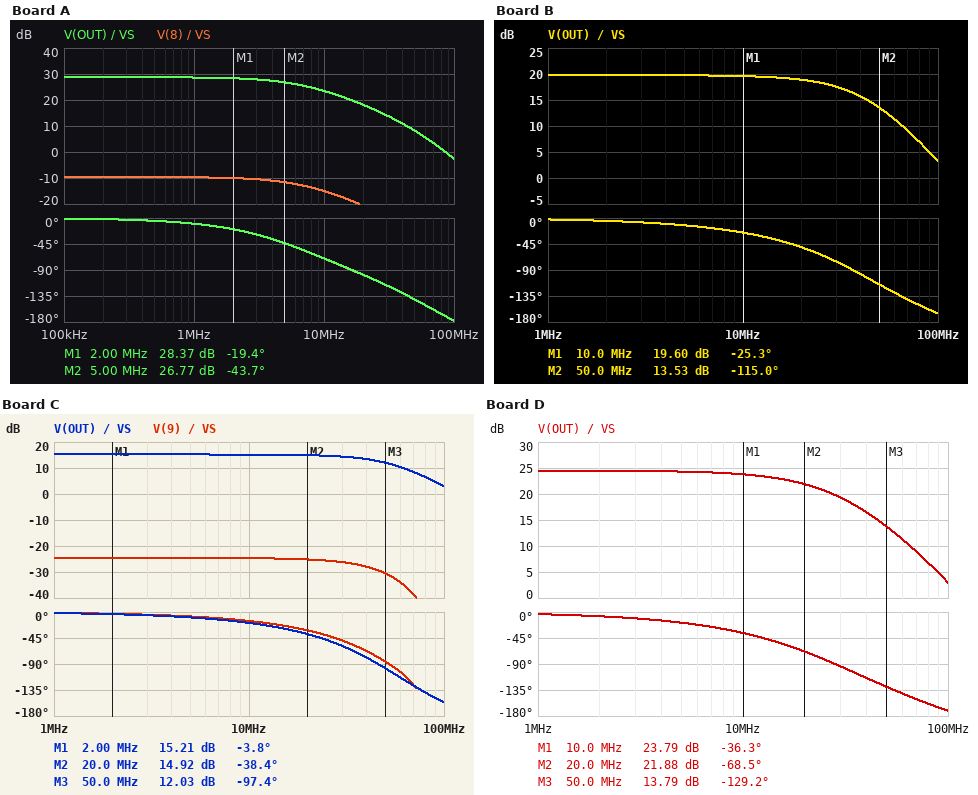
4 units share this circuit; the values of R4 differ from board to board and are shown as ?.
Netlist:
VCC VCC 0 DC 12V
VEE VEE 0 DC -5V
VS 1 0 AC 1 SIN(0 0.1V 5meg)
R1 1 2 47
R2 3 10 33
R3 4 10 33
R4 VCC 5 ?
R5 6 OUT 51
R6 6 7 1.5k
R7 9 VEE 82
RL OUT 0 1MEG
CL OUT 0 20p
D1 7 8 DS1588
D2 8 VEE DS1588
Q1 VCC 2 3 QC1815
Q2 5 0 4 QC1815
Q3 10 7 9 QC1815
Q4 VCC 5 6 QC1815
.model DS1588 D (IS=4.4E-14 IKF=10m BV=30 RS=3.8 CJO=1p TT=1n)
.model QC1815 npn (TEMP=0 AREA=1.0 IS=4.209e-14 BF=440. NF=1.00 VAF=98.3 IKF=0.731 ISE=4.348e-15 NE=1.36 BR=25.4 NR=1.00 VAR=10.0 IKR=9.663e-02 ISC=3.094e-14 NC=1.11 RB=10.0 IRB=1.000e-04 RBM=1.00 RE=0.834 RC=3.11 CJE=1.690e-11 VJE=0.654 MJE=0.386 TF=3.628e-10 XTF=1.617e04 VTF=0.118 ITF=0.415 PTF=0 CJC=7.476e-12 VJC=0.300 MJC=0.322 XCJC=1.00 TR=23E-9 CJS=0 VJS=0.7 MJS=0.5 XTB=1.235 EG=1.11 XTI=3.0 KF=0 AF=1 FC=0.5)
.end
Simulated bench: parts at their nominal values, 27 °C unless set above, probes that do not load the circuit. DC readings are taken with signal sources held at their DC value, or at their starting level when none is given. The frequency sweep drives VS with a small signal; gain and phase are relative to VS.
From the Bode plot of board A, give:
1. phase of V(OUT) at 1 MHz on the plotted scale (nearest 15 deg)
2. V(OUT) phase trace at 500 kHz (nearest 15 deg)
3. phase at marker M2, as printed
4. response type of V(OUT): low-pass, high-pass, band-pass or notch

-15 deg
0 deg
-43.7 deg
low-pass
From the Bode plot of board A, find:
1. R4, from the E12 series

3.3 kΩ
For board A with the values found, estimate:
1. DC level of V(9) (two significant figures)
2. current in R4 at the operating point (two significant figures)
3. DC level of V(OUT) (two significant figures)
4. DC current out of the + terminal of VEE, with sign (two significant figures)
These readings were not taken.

-4.4 V
3.6 mA
-430 mV
-9.4 mA
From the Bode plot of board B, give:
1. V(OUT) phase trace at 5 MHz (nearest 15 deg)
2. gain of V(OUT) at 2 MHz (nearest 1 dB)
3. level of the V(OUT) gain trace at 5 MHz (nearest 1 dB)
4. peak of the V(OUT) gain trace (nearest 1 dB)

-15 deg
20 dB
20 dB
20 dB
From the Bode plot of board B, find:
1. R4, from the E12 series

820 Ω
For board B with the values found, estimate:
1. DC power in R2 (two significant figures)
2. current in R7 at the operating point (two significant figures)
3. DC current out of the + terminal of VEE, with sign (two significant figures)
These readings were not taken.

620 µW
8.7 mA
-16 mA
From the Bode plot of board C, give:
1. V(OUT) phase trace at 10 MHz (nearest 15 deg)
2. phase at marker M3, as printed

-15 deg
-97.4 deg
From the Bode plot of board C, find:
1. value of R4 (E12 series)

470 Ω
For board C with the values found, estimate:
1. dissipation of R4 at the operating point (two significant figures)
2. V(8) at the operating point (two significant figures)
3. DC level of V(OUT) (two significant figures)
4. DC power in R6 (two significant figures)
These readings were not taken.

9.2 mW
-4.3 V
9.2 V
110 mW
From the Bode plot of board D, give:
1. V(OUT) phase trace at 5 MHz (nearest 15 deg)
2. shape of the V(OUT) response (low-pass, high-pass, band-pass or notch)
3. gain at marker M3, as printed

-15 deg
low-pass
13.79 dB
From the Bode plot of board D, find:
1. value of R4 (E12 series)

1.5 kΩ
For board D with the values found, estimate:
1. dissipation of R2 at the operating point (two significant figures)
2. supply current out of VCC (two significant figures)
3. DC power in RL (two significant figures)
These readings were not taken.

570 µW
14 mA
26 µW
